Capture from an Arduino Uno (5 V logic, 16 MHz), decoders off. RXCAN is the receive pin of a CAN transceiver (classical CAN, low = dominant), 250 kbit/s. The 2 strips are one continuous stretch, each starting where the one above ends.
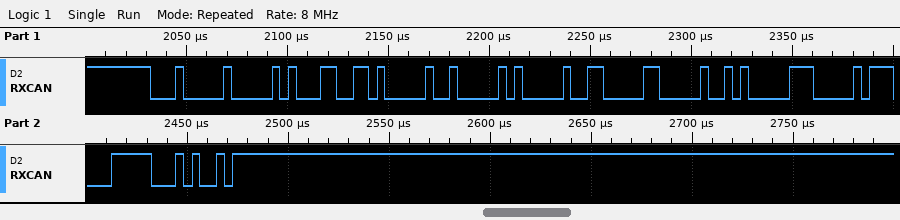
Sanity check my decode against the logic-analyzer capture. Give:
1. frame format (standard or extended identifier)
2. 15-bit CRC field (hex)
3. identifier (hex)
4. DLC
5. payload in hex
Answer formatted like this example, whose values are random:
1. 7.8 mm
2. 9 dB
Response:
1. standard
2. 0x0F94
3. 0x100
4. 8
5. CD 01 02 03 04 05 06 07
